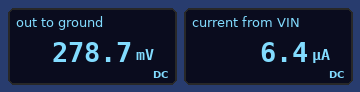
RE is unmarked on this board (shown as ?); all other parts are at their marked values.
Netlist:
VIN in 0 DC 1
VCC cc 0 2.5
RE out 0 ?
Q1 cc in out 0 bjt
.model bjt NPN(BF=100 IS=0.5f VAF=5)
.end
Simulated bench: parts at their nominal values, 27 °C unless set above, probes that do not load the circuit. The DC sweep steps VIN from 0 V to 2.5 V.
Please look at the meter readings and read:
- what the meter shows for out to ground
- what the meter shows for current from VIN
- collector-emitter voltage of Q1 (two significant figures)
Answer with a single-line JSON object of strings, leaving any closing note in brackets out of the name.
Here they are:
{"what the meter shows for out to ground": "278.7 mV", "what the meter shows for current from VIN": "6.4 µA", "collector-emitter voltage of Q1": "2.2 V"}
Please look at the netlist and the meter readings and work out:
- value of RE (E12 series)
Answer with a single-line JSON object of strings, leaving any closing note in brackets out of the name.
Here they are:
{"value of RE": "330 Ω"}
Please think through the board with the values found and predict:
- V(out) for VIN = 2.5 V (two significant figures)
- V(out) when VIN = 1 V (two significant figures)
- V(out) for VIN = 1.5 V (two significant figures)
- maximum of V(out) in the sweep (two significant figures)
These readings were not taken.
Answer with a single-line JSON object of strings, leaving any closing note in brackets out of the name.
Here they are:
{"V(out) for VIN = 2.5 V": "1.7 V", "V(out) when VIN = 1 V": "280 mV", "V(out) for VIN = 1.5 V": "750 mV", "maximum of V(out) in the sweep": "1.7 V"}
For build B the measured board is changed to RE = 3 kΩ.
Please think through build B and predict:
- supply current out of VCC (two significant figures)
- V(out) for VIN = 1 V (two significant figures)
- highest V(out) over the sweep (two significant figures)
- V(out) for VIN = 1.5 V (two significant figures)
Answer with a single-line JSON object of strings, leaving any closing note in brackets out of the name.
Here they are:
{"supply current out of VCC": "110 µA", "V(out) for VIN = 1 V": "330 mV", "highest V(out) over the sweep": "1.8 V", "V(out) for VIN = 1.5 V": "810 mV"}
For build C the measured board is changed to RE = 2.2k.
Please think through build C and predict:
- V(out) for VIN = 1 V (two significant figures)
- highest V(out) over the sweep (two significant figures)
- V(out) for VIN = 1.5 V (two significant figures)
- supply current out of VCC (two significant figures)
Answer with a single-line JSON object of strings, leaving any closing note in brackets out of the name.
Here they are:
{"V(out) for VIN = 1 V": "320 mV", "highest V(out) over the sweep": "1.8 V", "V(out) for VIN = 1.5 V": "800 mV", "supply current out of VCC": "150 µA"}
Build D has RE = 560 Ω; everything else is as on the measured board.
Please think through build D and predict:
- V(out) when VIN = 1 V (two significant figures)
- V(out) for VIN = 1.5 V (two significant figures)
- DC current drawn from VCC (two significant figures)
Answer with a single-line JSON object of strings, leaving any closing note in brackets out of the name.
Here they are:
{"V(out) when VIN = 1 V": "290 mV", "V(out) for VIN = 1.5 V": "760 mV", "DC current drawn from VCC": "520 µA"}
